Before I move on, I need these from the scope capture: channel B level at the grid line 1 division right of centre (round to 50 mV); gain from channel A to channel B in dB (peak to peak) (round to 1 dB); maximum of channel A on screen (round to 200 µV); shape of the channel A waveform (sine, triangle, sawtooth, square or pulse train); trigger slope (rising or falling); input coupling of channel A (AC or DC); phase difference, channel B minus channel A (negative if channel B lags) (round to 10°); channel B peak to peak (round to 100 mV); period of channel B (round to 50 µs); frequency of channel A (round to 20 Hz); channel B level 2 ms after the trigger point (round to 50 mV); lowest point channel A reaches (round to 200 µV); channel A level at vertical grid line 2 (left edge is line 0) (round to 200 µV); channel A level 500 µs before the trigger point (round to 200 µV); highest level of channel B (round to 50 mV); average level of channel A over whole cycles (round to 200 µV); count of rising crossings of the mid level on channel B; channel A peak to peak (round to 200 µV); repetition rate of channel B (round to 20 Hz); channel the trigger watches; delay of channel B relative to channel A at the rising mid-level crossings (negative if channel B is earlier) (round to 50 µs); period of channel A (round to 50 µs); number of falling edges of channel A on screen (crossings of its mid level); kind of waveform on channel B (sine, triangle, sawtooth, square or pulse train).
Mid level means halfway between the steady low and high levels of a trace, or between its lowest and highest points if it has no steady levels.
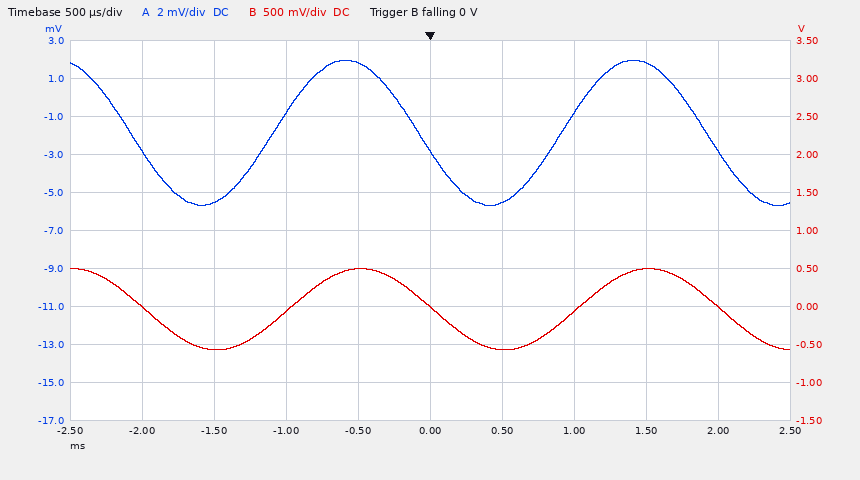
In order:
-550 mV
43 dB
2.0 mV
sine
falling
DC
-20°
1.10 V
2.00 ms
500 Hz
0 mV
-5.6 mV
-5.6 mV
1.8 mV
500 mV
-1.8 mV
2
7.6 mV
500 Hz
channel B
+100 µs
2.00 ms
3
sine
